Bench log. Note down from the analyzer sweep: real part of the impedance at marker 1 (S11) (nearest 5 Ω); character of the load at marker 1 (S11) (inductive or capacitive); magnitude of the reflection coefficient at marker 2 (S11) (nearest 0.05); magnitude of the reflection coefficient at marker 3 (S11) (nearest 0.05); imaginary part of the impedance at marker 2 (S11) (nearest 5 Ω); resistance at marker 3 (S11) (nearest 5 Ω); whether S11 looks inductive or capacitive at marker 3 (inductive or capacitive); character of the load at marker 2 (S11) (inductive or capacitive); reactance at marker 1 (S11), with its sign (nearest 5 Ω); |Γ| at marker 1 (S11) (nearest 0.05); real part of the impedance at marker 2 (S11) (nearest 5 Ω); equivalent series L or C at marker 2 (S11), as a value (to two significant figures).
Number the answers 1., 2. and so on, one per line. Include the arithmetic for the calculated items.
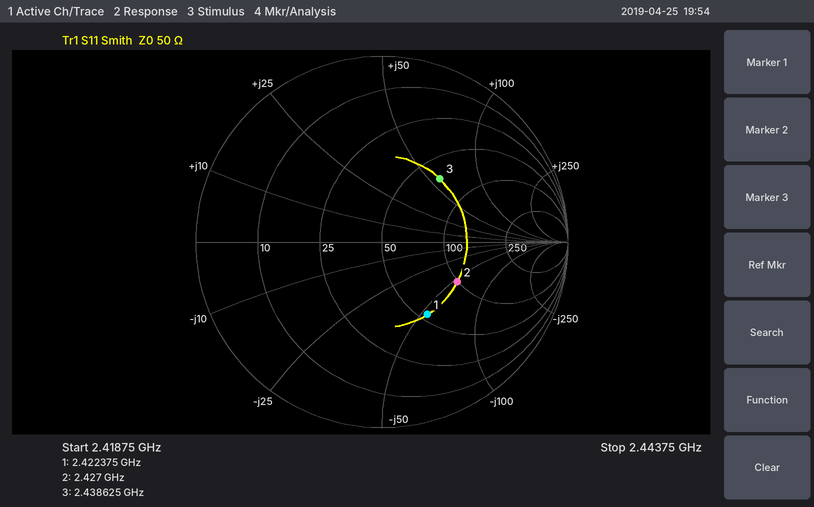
1. 55 Ω
2. capacitive
3. 0.45
4. 0.45
5. -55 Ω
6. 65 Ω
7. inductive
8. capacitive
9. -55 Ω
10. 0.45
11. 100 Ω
12. C = 1/(2π × 2.427 GHz × 55 Ω) ≈ 1.2 pF
